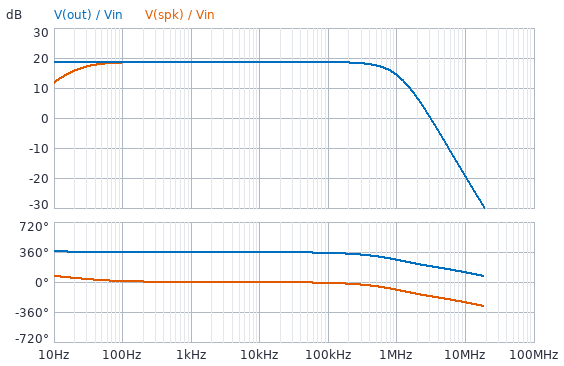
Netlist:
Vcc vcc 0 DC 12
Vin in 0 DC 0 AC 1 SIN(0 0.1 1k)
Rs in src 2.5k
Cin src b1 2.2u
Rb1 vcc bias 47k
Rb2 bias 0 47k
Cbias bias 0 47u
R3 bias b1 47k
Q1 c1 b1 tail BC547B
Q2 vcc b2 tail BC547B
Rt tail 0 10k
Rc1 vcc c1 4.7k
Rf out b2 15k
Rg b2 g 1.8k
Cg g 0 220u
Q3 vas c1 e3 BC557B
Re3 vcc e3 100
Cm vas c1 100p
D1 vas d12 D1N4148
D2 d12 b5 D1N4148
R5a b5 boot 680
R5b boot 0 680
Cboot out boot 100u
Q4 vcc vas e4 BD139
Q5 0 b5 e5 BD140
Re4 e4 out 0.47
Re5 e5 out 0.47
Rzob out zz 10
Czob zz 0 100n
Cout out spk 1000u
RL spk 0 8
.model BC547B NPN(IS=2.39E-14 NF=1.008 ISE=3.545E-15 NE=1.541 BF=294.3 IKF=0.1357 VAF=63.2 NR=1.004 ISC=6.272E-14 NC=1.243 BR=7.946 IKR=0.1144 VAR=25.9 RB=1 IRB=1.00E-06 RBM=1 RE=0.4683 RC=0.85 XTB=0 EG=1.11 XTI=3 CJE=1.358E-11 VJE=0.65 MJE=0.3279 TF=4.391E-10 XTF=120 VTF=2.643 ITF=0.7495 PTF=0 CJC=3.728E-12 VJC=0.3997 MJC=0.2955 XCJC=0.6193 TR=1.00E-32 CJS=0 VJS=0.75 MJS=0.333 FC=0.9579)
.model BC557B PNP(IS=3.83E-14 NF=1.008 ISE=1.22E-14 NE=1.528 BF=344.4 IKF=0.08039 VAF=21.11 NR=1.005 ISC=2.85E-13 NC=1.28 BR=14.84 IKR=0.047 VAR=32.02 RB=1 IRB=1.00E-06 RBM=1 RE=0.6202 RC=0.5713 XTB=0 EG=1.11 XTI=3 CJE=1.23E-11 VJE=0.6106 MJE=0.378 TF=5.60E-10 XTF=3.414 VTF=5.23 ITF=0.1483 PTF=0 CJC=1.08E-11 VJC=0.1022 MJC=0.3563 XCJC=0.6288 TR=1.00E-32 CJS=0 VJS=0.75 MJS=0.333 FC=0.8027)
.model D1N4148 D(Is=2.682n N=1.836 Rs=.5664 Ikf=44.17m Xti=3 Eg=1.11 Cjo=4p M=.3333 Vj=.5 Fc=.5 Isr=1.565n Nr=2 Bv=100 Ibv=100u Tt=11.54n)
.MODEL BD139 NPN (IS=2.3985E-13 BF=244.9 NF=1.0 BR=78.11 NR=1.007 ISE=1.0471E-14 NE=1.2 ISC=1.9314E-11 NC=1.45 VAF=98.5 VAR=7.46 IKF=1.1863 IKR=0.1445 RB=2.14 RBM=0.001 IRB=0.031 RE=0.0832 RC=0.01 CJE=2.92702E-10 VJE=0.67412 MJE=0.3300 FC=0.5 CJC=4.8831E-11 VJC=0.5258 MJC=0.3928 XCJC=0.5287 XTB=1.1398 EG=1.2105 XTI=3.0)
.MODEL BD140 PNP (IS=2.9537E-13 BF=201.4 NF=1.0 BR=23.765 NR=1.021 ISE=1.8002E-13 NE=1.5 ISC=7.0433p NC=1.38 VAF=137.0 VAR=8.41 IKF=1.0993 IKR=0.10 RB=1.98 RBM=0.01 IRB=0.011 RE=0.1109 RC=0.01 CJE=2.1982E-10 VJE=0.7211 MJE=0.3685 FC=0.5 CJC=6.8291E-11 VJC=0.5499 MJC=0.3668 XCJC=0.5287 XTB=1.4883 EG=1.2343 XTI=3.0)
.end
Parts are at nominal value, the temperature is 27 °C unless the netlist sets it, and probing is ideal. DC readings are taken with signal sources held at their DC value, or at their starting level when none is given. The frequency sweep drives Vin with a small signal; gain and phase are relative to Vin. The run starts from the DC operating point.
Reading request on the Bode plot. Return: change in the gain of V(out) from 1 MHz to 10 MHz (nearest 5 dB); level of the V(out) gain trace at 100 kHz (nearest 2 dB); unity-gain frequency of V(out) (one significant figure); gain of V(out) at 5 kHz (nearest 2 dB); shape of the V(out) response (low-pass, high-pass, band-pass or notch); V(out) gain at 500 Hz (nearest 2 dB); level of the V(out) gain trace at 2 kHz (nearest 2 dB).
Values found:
-35 dB
18 dB
3 MHz
18 dB
low-pass
18 dB
18 dB
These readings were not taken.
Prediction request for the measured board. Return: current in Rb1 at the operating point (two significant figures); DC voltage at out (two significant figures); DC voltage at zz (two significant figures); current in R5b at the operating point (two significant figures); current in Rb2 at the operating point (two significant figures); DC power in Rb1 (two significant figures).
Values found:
130 µA
6.0 V
6.0 V
3.9 mA
130 µA
770 µW
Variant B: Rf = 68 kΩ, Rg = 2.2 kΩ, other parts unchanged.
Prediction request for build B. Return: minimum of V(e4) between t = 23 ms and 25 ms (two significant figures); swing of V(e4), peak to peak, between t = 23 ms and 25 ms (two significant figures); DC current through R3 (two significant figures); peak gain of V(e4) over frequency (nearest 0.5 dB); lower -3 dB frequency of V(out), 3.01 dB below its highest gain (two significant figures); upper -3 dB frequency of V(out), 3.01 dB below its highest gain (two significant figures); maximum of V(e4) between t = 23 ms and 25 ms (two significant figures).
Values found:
3.5 V
5.3 V
770 nA
29.0 dB
1.8 Hz
180 kHz
8.8 V
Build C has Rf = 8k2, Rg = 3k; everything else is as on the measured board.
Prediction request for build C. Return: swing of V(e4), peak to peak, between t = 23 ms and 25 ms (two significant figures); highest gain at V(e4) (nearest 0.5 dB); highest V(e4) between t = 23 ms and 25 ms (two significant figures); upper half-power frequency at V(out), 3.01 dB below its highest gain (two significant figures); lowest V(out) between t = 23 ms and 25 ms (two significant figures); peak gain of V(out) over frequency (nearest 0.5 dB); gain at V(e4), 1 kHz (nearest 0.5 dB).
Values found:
730 mV
13.0 dB
6.3 V
1.9 MHz
5.6 V
12.5 dB
11.0 dB
